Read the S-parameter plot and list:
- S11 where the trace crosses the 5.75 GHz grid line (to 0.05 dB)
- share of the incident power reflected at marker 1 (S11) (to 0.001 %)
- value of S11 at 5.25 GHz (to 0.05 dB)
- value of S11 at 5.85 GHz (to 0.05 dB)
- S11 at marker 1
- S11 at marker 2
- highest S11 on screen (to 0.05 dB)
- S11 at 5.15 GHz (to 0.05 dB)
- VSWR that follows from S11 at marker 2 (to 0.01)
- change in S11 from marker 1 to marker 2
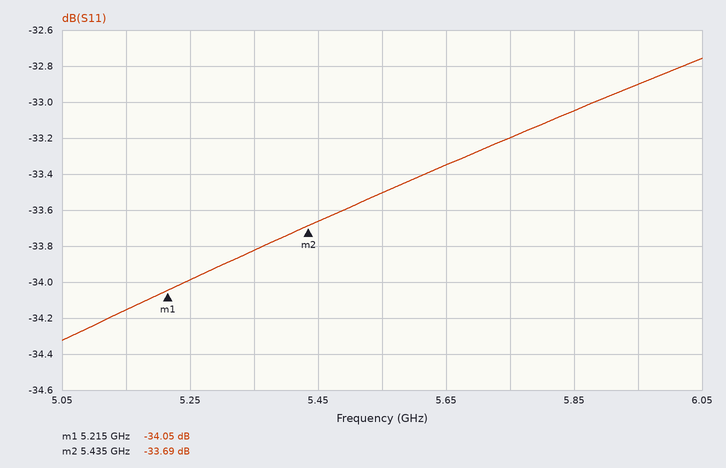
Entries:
-33.20 dB
0.039 %
-34.00 dB
-33.05 dB
-34.05 dB
-33.69 dB
-32.75 dB
-34.15 dB
1.04
0.36 dB
